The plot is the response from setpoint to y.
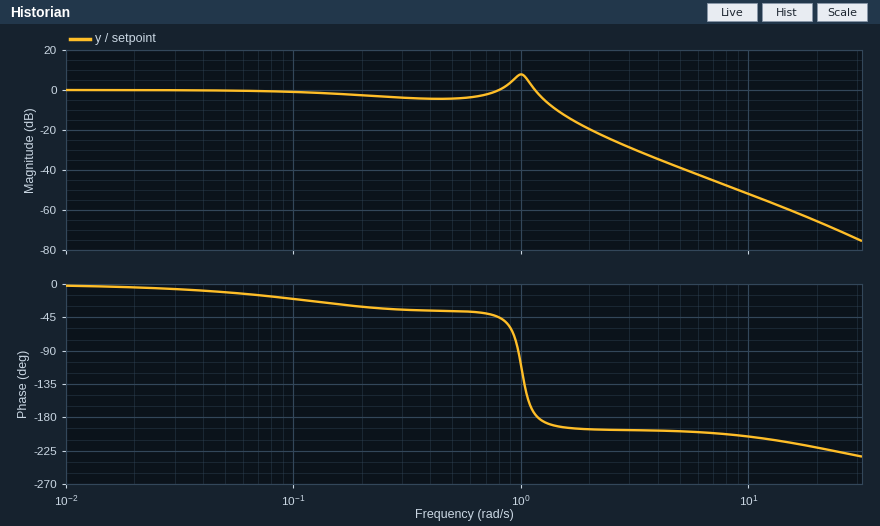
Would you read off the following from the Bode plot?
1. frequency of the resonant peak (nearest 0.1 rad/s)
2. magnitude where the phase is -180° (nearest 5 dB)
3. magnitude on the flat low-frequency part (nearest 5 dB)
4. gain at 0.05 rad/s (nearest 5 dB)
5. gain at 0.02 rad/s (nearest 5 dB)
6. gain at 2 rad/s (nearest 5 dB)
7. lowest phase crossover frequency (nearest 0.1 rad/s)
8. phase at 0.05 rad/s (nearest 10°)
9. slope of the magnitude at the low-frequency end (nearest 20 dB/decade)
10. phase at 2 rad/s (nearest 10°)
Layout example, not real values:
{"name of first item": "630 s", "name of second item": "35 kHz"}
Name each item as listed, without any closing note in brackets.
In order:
{"frequency of the resonant peak": "1.0 rad/s", "magnitude where the phase is -180°": "0 dB", "magnitude on the flat low-frequency part": "0 dB", "gain at 0.05 rad/s": "0 dB", "gain at 0.02 rad/s": "0 dB", "gain at 2 rad/s": "-20 dB", "lowest phase crossover frequency": "1.2 rad/s", "phase at 0.05 rad/s": "-10°", "slope of the magnitude at the low-frequency end": "0 dB/decade", "phase at 2 rad/s": "-200°"}
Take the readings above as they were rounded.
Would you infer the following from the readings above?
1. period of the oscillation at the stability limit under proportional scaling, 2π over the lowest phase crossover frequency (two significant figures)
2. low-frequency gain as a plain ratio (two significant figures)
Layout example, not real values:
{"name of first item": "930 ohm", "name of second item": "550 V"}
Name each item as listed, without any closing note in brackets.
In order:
{"period of the oscillation at the stability limit under proportional scaling, 2π over the lowest phase crossover frequency": "5.2 s", "low-frequency gain as a plain ratio": "1.0"}
